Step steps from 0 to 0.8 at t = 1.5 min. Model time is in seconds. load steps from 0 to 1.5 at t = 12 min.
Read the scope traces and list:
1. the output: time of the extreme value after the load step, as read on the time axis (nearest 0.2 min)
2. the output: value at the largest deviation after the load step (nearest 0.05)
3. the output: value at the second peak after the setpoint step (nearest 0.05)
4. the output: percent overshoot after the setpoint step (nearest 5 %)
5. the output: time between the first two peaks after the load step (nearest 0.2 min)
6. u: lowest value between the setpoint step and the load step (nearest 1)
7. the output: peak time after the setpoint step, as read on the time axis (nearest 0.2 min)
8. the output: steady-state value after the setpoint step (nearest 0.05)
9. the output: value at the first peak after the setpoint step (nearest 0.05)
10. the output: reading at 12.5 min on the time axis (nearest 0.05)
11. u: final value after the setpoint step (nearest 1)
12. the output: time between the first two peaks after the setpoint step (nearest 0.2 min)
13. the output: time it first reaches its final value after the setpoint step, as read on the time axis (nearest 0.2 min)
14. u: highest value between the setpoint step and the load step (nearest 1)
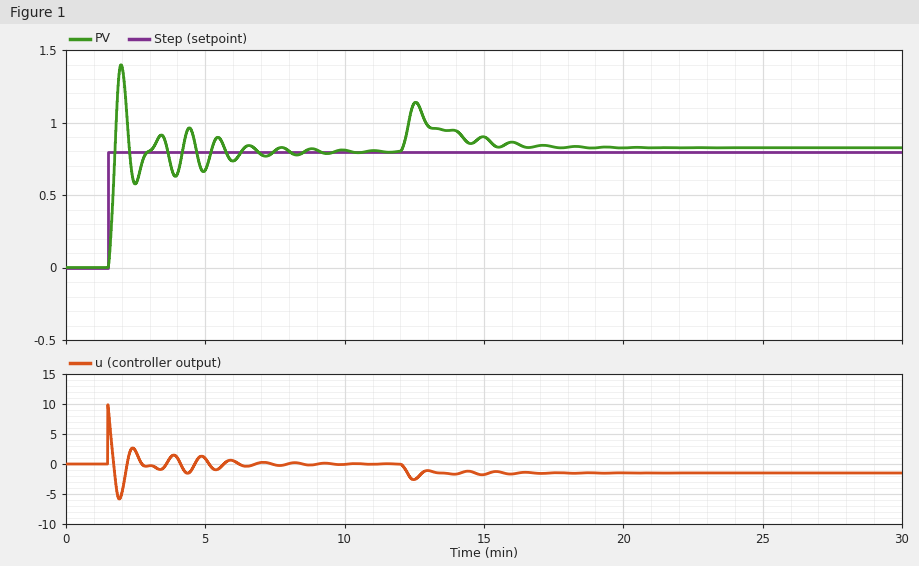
12.6 min
1.15
0.90
75 %
2.4 min
-6
2.0 min
0.80
1.40
1.15
0
1.4 min
1.8 min
10
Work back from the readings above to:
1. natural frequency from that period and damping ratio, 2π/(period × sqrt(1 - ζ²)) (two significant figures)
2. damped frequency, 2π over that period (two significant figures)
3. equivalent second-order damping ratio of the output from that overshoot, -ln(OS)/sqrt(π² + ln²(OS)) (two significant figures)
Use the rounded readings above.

4.5 rad/min
4.5 rad/min
0.091
